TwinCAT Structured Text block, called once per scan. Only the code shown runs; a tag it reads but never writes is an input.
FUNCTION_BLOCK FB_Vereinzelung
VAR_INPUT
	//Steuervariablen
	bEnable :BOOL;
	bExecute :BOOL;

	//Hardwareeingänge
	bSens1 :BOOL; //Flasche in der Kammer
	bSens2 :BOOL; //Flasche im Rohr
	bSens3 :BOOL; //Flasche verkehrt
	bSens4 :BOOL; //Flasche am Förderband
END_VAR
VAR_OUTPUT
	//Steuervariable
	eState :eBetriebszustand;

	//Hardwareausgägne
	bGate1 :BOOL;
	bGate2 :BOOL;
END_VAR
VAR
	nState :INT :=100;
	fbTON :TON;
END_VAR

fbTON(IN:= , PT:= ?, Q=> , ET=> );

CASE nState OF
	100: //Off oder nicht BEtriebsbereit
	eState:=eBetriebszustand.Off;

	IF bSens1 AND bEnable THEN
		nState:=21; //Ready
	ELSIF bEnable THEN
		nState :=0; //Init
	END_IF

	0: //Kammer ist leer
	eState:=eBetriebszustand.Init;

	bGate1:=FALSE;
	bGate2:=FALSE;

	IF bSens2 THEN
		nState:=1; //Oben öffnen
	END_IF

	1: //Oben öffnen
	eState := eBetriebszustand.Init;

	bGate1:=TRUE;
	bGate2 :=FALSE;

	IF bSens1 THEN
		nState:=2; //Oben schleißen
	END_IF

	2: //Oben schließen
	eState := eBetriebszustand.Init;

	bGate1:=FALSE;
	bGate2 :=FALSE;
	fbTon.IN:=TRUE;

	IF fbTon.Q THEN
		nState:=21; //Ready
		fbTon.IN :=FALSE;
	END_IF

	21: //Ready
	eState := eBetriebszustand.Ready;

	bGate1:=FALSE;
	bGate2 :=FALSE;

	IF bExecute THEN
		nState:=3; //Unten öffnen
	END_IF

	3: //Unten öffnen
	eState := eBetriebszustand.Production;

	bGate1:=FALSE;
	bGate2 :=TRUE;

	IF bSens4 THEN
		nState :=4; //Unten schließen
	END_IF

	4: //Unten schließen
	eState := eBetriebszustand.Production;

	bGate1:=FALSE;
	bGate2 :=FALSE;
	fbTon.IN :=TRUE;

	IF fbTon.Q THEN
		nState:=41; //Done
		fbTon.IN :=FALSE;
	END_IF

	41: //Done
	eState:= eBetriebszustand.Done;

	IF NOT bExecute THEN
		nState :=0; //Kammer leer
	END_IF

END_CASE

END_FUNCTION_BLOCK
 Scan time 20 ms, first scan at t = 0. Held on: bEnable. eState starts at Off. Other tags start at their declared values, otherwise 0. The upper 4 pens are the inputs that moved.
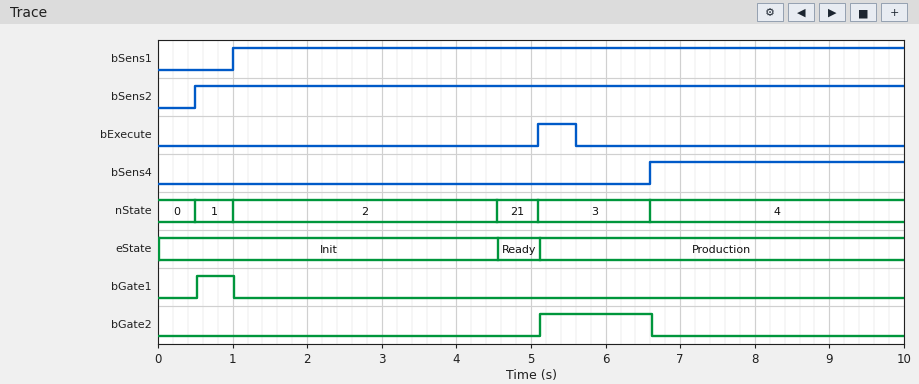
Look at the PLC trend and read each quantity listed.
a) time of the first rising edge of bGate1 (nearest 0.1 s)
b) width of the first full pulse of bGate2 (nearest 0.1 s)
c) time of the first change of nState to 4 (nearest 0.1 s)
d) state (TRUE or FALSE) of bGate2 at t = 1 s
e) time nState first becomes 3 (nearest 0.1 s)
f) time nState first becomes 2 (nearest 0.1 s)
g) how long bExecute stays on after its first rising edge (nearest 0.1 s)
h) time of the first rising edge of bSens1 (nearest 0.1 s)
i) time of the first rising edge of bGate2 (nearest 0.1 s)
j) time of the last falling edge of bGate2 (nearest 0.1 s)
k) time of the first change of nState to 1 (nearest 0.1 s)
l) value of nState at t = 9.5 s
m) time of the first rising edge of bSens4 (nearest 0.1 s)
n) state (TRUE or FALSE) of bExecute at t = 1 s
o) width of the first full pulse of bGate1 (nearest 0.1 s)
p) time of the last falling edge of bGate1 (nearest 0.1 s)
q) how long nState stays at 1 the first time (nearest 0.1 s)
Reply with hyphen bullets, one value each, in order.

- 0.5 s
- 1.5 s
- 6.6 s
- FALSE
- 5.1 s
- 1.0 s
- 0.5 s
- 1.0 s
- 5.1 s
- 6.6 s
- 0.5 s
- 4
- 6.6 s
- FALSE
- 0.5 s
- 1.0 s
- 0.5 s
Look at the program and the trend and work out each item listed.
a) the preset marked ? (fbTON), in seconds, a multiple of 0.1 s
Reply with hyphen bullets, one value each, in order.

- 3.5 s
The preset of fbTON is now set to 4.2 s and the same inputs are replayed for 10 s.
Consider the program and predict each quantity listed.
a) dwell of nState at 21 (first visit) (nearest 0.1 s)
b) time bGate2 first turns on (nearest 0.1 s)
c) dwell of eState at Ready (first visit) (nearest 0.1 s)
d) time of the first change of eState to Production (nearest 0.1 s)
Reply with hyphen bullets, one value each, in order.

- 0.0 s
- 5.3 s
- 0.0 s
- 5.3 s
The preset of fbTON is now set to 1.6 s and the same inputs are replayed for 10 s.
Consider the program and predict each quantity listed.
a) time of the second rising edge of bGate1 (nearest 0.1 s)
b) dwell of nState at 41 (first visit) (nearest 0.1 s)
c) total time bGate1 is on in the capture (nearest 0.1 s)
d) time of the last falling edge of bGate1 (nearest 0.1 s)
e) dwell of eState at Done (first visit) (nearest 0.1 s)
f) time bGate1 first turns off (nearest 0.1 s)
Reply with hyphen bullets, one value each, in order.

- 8.3 s
- 0.0 s
- 0.5 s
- 8.3 s
- 0.0 s
- 1.0 s
